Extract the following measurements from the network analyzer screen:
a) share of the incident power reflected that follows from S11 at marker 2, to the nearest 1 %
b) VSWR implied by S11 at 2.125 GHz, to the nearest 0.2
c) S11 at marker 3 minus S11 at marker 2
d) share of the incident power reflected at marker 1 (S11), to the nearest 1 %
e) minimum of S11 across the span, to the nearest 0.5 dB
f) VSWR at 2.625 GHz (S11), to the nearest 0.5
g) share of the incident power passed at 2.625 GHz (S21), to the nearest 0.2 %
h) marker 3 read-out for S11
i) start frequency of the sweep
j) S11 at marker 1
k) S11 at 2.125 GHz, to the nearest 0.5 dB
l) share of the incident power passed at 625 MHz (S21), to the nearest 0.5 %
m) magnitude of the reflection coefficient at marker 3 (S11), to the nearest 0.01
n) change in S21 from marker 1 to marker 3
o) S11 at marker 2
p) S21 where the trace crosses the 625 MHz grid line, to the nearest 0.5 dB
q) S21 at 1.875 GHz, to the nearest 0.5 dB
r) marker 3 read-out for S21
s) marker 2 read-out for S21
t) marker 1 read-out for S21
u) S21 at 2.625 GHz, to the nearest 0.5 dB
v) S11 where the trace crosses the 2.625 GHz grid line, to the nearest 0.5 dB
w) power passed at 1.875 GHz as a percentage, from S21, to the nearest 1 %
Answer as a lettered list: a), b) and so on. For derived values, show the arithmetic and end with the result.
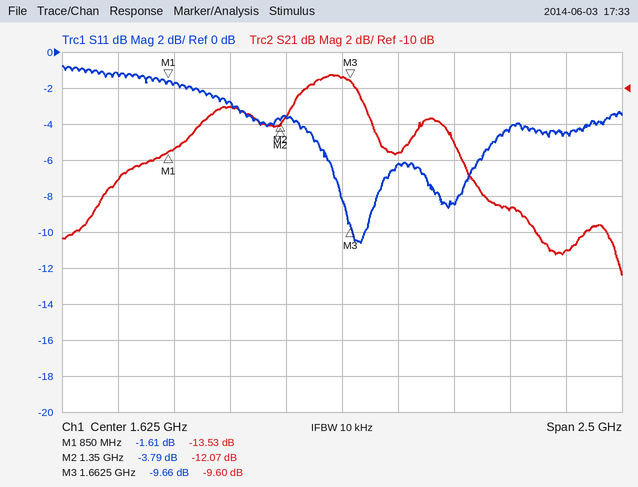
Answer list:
a) 10^(-3.79/10) ≈ 42 %
b) |Γ| = 10^(-8.5/20) = 0.3758; VSWR = (1 + 0.3758)/(1 − 0.3758) ≈ 2.2
c) -9.66 − (-3.79) = -5.87 dB
d) 10^(-1.61/10) ≈ 69 %
e) -10.5 dB
f) |Γ| = 10^(-4.5/20) = 0.5957; VSWR = (1 + 0.5957)/(1 − 0.5957) ≈ 4.0
g) 10^(-19/10) ≈ 1.26 %, so 1.2 % to the nearest 0.2 %
h) -9.66 dB
i) 375 MHz
j) -1.61 dB
k) -8.5 dB
l) 10^(-15/10) ≈ 3.16 %, so 3.0 % to the nearest 0.5 %
m) 10^(-9.66/20) ≈ 0.33
n) -9.6 − (-13.53) = 3.93 dB
o) -3.79 dB
p) -15.0 dB
q) -13.5 dB
r) -9.60 dB
s) -12.07 dB
t) -13.53 dB
u) -19.0 dB
v) -4.5 dB
w) 10^(-13.5/10) ≈ 4 %
